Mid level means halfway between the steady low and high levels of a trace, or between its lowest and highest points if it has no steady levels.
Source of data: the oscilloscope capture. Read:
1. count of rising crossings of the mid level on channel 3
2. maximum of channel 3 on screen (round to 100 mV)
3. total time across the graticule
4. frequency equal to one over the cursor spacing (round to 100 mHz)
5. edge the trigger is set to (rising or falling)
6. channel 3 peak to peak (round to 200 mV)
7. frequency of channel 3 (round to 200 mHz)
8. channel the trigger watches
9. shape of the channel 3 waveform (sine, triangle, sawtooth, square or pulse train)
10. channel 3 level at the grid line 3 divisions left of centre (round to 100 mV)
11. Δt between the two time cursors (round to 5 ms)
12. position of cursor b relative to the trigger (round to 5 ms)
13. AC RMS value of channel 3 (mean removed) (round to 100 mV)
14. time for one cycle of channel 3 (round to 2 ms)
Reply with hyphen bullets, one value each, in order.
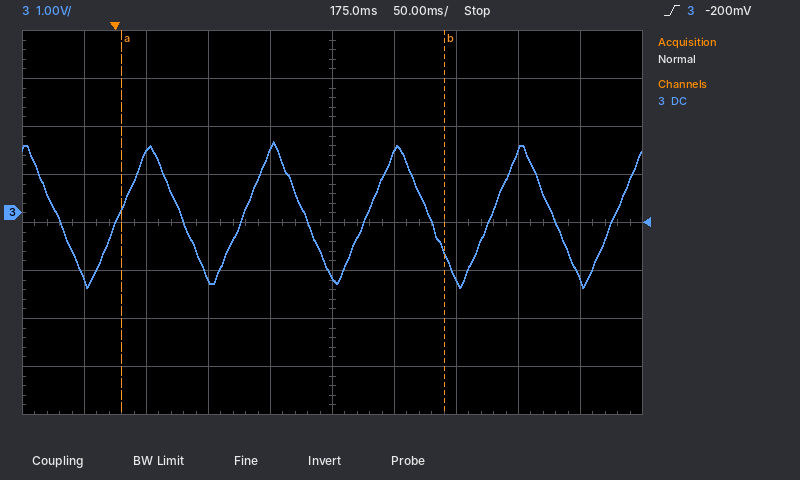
- 5
- 1.5 V
- 500 ms
- 3.8 Hz
- rising
- 3.0 V
- 10.0 Hz
- channel 3
- triangle
- 1.3 V
- 260 ms
- +265 ms
- 900 mV
- 100 ms
